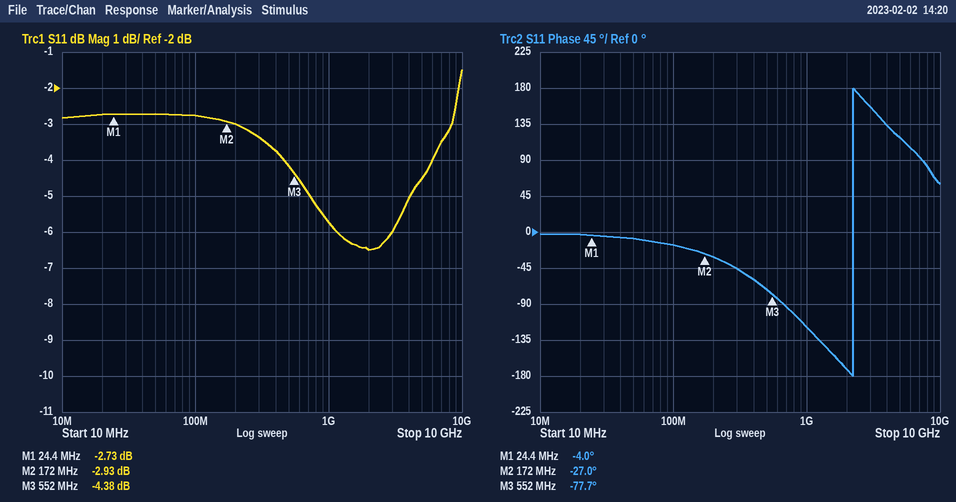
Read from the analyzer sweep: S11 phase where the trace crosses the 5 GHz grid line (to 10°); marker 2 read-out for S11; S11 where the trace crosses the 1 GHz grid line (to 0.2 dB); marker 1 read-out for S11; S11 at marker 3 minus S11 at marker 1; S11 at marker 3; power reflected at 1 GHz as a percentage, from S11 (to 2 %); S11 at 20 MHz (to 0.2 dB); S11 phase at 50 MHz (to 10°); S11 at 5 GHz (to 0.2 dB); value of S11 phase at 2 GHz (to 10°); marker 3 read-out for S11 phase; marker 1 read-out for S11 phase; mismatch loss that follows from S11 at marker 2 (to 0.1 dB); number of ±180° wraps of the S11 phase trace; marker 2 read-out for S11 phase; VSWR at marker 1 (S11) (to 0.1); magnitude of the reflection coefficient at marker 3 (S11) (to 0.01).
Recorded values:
120°
-2.93 dB
-5.8 dB
-2.73 dB
-1.65 dB
-4.38 dB
26 %
-2.8 dB
-10°
-4.6 dB
-170°
-77.7°
-4.0°
3.1 dB
1
-27.0°
6.4
0.60
